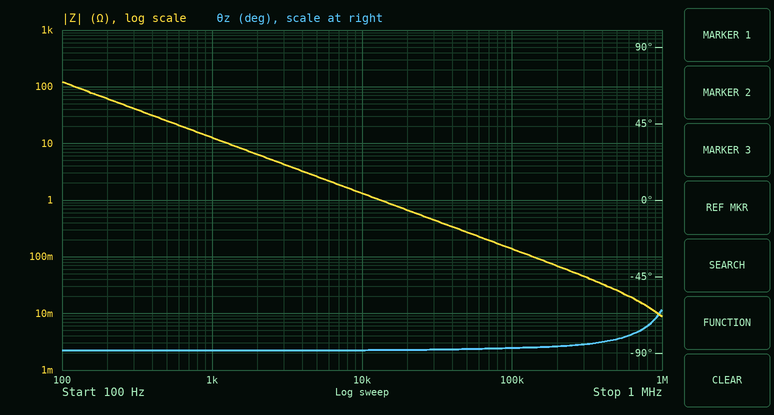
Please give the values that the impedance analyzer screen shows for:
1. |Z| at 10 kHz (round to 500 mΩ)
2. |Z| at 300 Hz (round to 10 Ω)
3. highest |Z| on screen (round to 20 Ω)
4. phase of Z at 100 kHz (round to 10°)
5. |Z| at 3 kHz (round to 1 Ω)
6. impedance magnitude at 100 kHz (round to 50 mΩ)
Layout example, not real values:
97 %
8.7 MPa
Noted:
1.5 Ω
40 Ω
120 Ω
-90°
4 Ω
150 mΩ
